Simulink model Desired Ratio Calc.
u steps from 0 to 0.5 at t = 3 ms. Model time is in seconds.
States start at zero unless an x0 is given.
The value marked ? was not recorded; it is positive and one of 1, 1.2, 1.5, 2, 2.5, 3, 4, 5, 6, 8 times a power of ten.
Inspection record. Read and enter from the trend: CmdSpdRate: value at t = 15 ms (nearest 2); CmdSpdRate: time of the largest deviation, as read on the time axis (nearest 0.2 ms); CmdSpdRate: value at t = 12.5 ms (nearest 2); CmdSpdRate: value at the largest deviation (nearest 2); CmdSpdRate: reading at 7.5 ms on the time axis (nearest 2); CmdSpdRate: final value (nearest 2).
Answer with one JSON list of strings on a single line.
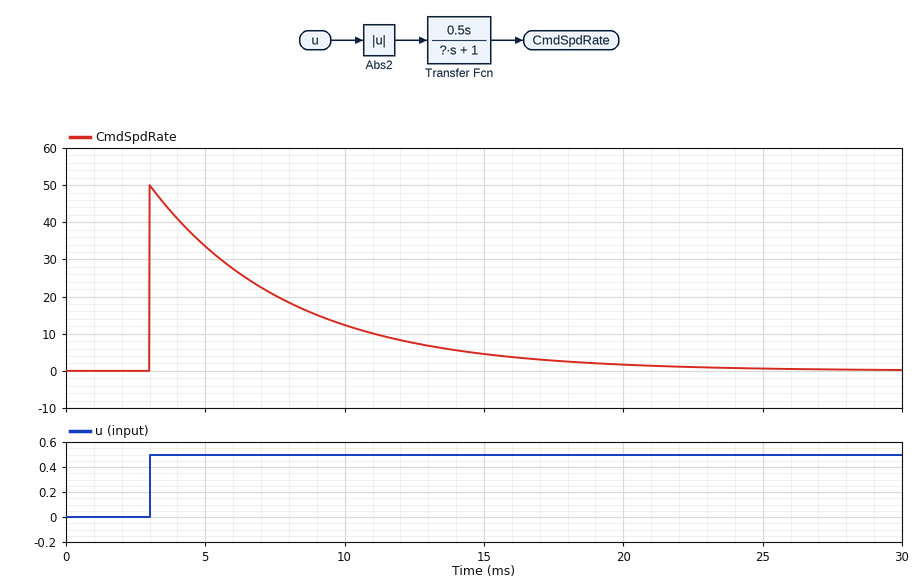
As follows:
["4", "3.0 ms", "8", "50", "20", "0"]
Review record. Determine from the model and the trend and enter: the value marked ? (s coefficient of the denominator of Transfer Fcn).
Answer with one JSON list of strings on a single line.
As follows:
["0.005"]
